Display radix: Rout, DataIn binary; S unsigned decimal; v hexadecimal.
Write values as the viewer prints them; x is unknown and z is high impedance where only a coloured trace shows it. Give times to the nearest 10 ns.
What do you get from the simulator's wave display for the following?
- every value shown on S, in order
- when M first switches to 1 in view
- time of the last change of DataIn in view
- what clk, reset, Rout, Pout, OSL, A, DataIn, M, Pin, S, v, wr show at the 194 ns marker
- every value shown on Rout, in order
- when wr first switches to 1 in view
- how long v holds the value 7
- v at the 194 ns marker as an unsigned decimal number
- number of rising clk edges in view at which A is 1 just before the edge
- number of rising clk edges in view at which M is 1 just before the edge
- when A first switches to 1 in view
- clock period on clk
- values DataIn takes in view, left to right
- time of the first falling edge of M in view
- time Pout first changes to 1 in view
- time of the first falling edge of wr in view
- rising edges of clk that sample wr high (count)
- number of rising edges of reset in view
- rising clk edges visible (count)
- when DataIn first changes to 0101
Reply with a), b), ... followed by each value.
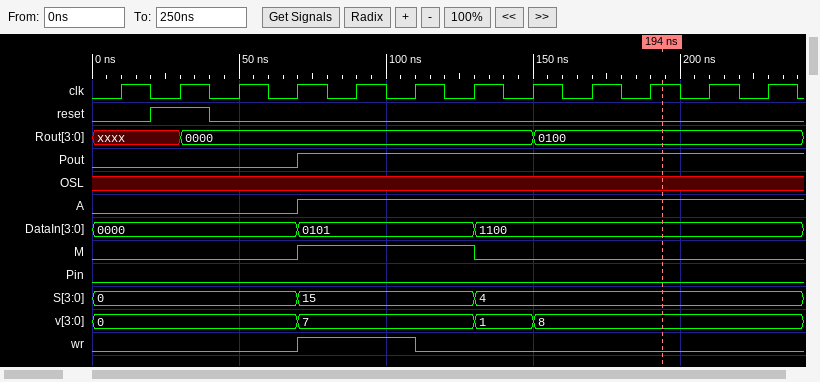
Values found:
a) 0, 15, 4
b) 70 ns
c) 130 ns
d) clk=1, reset=0, Rout=0100, Pout=1, OSL=x, A=1, DataIn=1100, M=0, Pin=0, S=4, v=8, wr=0
e) xxxx, 0000, 0100
f) 70 ns
g) 60 ns
h) 8
i) 8
j) 3
k) 70 ns
l) 20 ns
m) 0000, 0101, 1100
n) 130 ns
o) 70 ns
p) 110 ns
q) 2
r) 1
s) 12
t) 70 ns
